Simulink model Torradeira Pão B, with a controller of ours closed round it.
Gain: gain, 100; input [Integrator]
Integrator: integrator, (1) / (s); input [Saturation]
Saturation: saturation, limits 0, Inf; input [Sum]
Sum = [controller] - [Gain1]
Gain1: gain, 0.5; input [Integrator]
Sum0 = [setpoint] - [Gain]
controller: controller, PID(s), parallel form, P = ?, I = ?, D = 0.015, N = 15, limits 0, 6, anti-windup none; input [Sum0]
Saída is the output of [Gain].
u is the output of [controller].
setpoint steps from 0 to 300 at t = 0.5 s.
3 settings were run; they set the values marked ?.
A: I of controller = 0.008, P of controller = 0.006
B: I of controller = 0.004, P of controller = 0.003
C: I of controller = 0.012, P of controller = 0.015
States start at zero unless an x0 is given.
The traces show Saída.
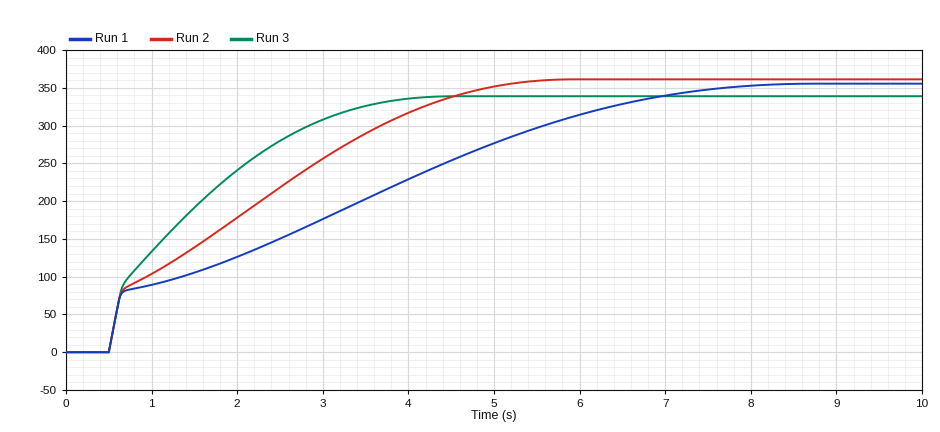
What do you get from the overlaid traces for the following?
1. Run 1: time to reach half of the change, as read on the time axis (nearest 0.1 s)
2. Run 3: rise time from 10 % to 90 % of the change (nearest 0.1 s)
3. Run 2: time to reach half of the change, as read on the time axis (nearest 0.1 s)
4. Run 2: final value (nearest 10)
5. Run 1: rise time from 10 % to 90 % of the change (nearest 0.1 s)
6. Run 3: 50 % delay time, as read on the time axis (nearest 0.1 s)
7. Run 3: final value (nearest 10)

3.0 s
2.4 s
2.0 s
360
5.6 s
1.3 s
340
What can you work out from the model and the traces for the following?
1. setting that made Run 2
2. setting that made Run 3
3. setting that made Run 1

A
C
B
